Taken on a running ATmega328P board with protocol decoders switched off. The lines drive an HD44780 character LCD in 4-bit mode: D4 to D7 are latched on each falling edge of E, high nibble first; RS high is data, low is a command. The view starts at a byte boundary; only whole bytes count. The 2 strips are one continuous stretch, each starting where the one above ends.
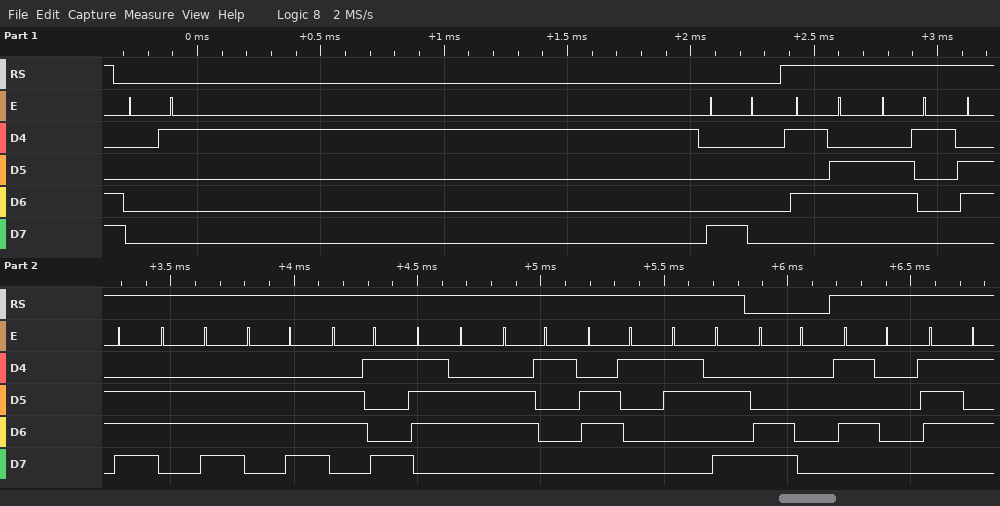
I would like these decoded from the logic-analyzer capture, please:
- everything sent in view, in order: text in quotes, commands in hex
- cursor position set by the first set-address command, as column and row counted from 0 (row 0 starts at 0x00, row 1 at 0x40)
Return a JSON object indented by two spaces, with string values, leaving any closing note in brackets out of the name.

{
  "everything sent in view, in order: text in quotes, commands in hex": "0x01 0x80 \"Vannnivaa:\" 0xC0 \"Pu\"",
  "cursor position set by the first set-address command, as column and row counted from 0": "column 0, row 0"
}
